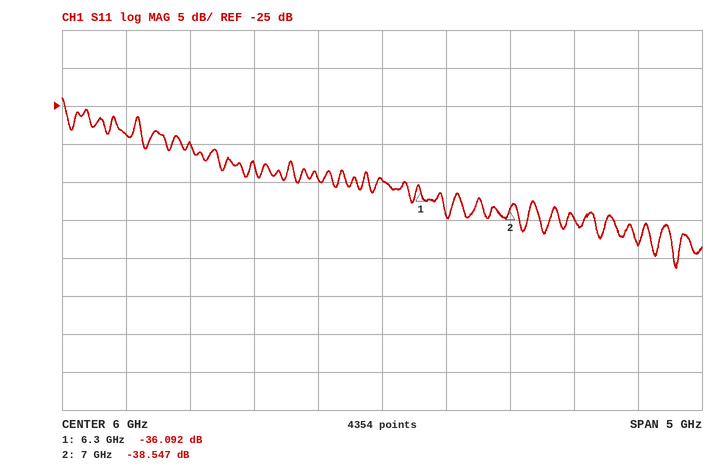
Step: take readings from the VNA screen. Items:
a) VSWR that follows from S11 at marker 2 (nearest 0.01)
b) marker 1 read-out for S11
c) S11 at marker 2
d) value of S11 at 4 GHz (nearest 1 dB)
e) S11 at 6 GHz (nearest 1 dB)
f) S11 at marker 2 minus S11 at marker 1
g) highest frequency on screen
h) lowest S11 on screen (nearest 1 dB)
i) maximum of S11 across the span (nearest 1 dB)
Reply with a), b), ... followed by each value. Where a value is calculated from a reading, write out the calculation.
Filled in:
a) (1 + 0.0118)/(1 − 0.0118) ≈ 1.02
b) -36.092 dB
c) -38.547 dB
d) -29 dB
e) -35 dB
f) -38.547 − (-36.092) = -2.455 dB
g) 8.5 GHz
h) -46 dB
i) -24 dB
